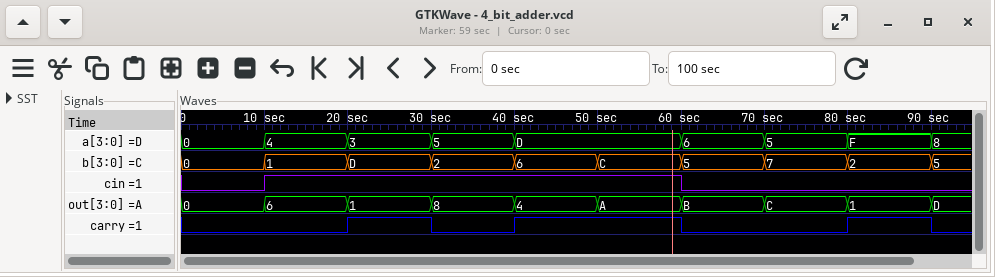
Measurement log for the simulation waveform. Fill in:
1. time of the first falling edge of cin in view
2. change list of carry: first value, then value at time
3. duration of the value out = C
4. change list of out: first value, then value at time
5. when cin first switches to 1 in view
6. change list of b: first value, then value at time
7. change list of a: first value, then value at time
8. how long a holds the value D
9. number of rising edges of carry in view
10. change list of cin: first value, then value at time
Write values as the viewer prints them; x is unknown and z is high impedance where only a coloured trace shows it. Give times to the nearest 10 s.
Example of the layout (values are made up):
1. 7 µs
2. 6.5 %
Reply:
1. 60 s
2. 0, 1 at 20 s, 0 at 30 s, 1 at 40 s, 0 at 60 s, 1 at 80 s, 0 at 90 s
3. 10 s
4. 0, 6 at 10 s, 1 at 20 s, 8 at 30 s, 4 at 40 s, A at 50 s, B at 60 s, C at 70 s, 1 at 80 s, D at 90 s
5. 10 s
6. 0, 1 at 10 s, D at 20 s, 2 at 30 s, 6 at 40 s, C at 50 s, 5 at 60 s, 7 at 70 s, 2 at 80 s, 5 at 90 s
7. 0, 4 at 10 s, 3 at 20 s, 5 at 30 s, D at 40 s, 6 at 60 s, 5 at 70 s, F at 80 s, 8 at 90 s
8. 20 s
9. 3
10. 0, 1 at 10 s, 0 at 60 s
